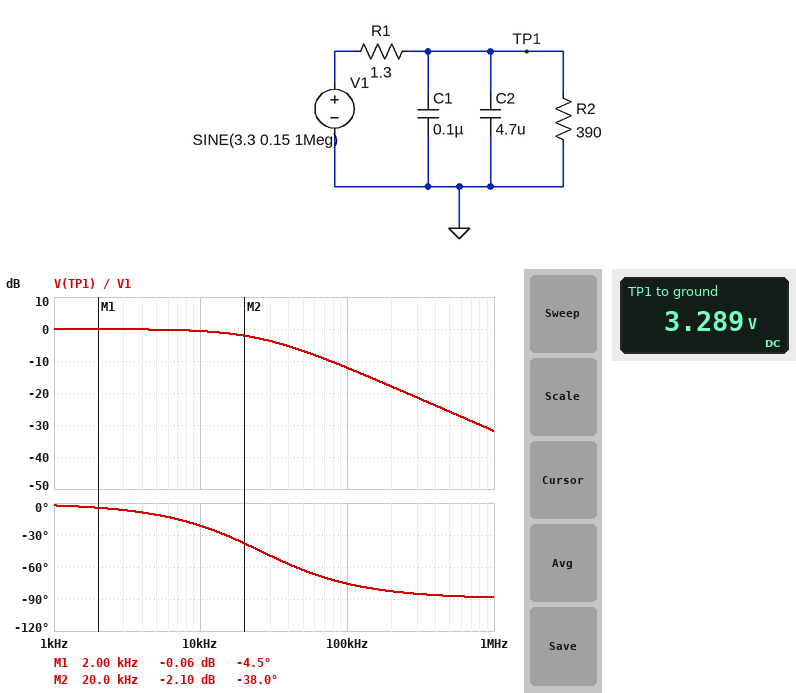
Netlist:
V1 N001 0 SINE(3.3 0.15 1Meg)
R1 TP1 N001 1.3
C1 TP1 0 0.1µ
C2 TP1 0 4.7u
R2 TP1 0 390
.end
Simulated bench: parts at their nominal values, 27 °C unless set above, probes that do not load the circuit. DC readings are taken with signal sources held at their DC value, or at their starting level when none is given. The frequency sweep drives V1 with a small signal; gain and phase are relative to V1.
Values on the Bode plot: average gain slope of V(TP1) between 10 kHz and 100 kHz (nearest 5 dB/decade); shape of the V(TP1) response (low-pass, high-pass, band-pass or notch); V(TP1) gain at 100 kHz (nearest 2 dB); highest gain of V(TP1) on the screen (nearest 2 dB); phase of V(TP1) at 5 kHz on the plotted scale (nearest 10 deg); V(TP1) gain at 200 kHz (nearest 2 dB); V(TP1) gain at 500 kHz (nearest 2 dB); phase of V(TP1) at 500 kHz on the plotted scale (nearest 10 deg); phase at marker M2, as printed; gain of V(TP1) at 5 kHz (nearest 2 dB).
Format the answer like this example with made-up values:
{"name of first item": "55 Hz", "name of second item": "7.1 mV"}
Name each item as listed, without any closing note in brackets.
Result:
{"average gain slope of V(TP1) between 10 kHz and 100 kHz": "-10 dB/decade", "shape of the V(TP1) response": "low-pass", "V(TP1) gain at 100 kHz": "-12 dB", "highest gain of V(TP1) on the screen": "0 dB", "phase of V(TP1) at 5 kHz on the plotted scale": "-10 deg", "V(TP1) gain at 200 kHz": "-18 dB", "V(TP1) gain at 500 kHz": "-26 dB", "phase of V(TP1) at 500 kHz on the plotted scale": "-90 deg", "phase at marker M2, as printed": "-38.0 deg", "gain of V(TP1) at 5 kHz": "0 dB"}
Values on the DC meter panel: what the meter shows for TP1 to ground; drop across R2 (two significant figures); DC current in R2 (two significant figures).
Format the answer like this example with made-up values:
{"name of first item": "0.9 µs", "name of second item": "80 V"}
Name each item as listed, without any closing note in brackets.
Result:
{"what the meter shows for TP1 to ground": "3.289 V", "drop across R2": "3.3 V", "DC current in R2": "8.4 mA"}
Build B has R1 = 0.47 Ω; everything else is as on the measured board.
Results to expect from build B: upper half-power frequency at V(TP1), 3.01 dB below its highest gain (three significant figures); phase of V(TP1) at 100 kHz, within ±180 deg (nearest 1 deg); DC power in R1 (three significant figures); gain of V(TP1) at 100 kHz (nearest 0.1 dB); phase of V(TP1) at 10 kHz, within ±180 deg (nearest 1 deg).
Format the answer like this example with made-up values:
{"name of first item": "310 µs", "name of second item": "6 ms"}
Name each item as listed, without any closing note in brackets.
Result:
{"upper half-power frequency at V(TP1), 3.01 dB below its highest gain": "70.6 kHz", "phase of V(TP1) at 100 kHz, within ±180 deg": "-55 deg", "DC power in R1": "33.6 µW", "gain of V(TP1) at 100 kHz": "-4.8 dB", "phase of V(TP1) at 10 kHz, within ±180 deg": "-8 deg"}
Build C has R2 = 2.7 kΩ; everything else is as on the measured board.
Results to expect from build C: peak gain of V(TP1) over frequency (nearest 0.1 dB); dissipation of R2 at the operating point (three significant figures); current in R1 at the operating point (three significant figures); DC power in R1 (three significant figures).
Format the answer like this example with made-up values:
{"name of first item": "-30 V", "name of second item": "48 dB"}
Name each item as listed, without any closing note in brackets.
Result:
{"peak gain of V(TP1) over frequency": "0 dB", "dissipation of R2 at the operating point": "4.03 mW", "current in R1 at the operating point": "1.22 mA", "DC power in R1": "1.94 µW"}
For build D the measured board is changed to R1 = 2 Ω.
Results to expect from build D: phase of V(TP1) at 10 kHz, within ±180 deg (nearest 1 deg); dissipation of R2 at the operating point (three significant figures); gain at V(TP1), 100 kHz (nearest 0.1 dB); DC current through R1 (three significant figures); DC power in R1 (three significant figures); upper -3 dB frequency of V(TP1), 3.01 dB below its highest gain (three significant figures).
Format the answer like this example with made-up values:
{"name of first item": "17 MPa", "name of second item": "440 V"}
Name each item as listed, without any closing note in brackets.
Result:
{"phase of V(TP1) at 10 kHz, within ±180 deg": "-31 deg", "dissipation of R2 at the operating point": "27.6 mW", "gain at V(TP1), 100 kHz": "-15.7 dB", "DC current through R1": "8.42 mA", "DC power in R1": "142 µW", "upper -3 dB frequency of V(TP1), 3.01 dB below its highest gain": "16.7 kHz"}
